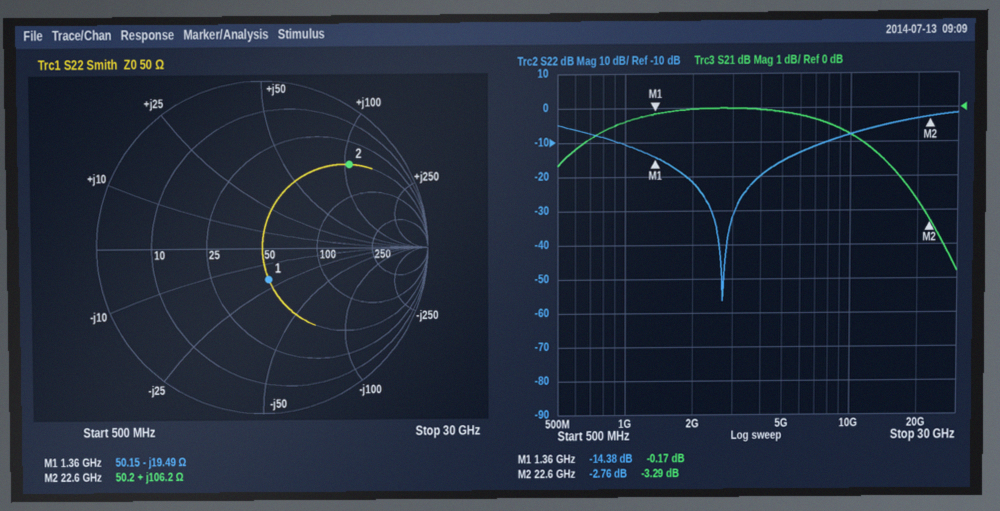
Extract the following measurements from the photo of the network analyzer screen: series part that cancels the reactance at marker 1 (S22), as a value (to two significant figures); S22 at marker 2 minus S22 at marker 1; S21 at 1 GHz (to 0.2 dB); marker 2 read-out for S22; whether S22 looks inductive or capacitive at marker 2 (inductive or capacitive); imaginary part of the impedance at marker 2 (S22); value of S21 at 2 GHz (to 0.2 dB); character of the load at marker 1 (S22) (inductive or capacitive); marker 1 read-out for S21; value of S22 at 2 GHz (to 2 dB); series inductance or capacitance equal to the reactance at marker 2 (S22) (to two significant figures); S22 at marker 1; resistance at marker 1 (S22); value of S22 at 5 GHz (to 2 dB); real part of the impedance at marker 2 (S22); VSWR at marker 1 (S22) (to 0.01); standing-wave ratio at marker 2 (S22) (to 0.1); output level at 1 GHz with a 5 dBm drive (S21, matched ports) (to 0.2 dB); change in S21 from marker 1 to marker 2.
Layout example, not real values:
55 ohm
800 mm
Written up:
2.3 nH
11.62 dB
-0.4 dB
-2.76 dB
inductive
+106.2 Ω
0.0 dB
capacitive
-0.17 dB
-22 dB
750 pH
-14.38 dB
50.15 Ω
-16 dB
50.2 Ω
1.47
6.3
4.6 dBm
-3.12 dB
